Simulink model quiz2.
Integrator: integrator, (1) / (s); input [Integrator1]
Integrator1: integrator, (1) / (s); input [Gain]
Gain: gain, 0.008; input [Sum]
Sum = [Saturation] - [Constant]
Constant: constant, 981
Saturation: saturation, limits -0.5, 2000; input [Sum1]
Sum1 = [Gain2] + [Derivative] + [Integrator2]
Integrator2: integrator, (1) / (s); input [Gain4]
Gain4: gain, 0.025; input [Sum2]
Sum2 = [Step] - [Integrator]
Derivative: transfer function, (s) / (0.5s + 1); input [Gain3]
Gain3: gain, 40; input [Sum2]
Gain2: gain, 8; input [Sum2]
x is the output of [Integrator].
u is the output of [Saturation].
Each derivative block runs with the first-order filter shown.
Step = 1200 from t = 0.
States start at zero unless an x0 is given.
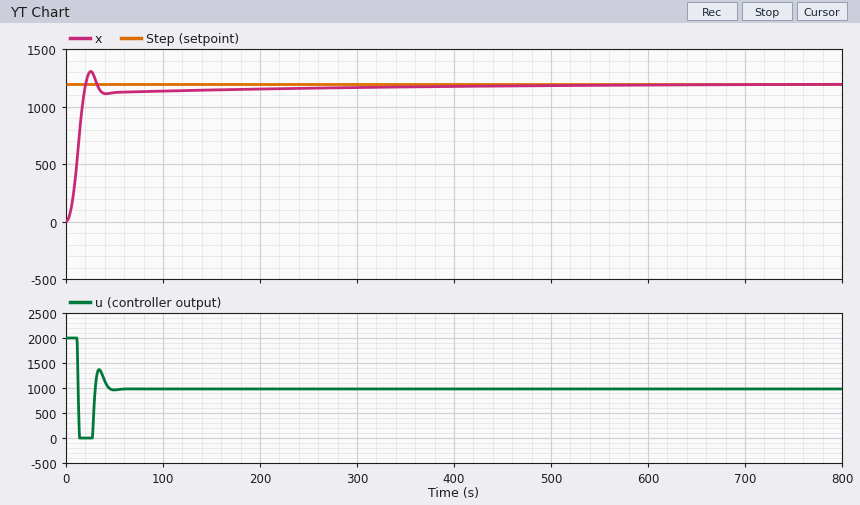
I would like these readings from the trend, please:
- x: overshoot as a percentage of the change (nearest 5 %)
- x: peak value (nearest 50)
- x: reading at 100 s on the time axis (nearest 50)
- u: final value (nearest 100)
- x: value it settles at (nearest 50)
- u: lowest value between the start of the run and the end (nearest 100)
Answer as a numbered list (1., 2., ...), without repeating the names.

1. 10 %
2. 1300
3. 1150
4. 1000
5. 1200
6. 0
